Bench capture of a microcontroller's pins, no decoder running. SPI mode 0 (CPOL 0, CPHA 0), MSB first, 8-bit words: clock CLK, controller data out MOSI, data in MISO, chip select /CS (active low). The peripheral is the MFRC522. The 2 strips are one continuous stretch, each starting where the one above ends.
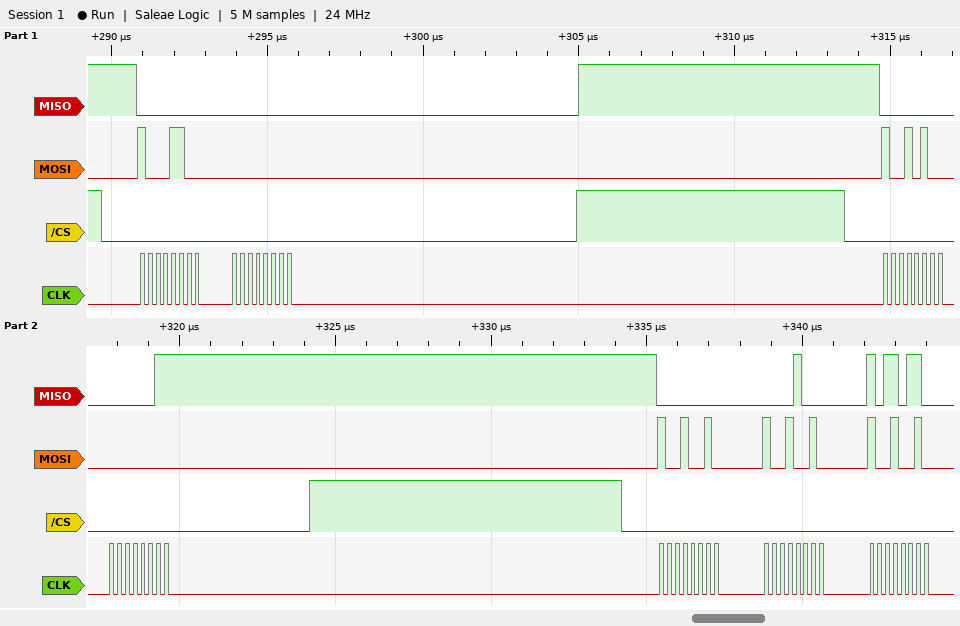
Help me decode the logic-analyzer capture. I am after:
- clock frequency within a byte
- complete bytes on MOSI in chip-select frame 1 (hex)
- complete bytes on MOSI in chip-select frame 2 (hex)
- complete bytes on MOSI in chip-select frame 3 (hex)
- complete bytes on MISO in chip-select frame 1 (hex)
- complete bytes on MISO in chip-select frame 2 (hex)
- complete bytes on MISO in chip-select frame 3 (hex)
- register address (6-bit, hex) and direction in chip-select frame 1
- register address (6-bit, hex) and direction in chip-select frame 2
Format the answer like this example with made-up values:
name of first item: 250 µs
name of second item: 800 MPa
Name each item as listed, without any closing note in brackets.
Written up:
clock frequency within a byte: 4 MHz
complete bytes on MOSI in chip-select frame 1: 8C 00
complete bytes on MOSI in chip-select frame 2: 94 00
complete bytes on MOSI in chip-select frame 3: 92 92 92
complete bytes on MISO in chip-select frame 1: 00 00
complete bytes on MISO in chip-select frame 2: 00 03
complete bytes on MISO in chip-select frame 3: 00 08 B6
register address (6-bit, hex) and direction in chip-select frame 1: 0x06 read
register address (6-bit, hex) and direction in chip-select frame 2: 0x0A read
